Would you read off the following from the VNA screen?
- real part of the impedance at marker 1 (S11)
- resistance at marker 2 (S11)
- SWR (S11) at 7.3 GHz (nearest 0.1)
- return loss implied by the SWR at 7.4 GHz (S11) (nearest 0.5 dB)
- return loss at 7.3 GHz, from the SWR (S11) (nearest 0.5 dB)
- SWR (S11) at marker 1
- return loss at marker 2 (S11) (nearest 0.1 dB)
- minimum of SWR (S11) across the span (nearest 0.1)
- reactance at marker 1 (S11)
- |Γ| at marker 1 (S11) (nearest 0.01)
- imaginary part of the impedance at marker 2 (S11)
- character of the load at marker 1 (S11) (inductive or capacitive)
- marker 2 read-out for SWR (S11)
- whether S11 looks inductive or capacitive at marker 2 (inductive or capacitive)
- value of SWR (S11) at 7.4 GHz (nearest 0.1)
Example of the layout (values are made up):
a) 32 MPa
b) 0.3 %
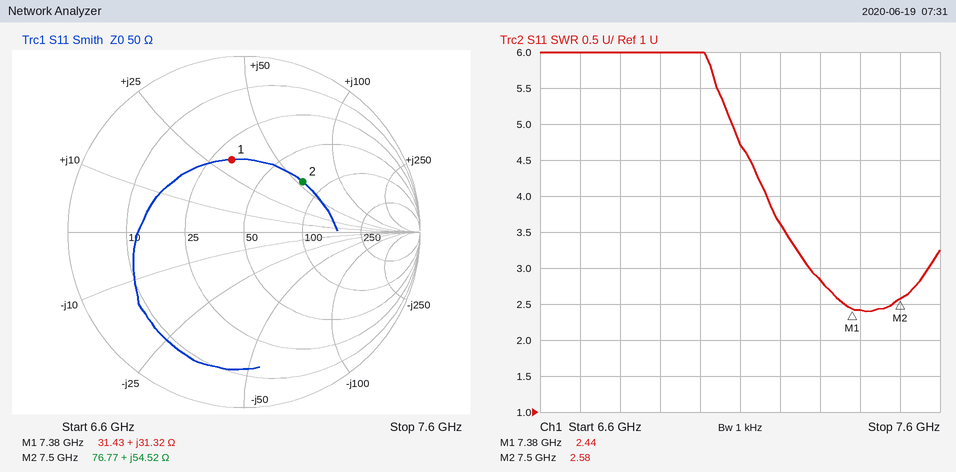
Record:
a) 31.43 Ω
b) 76.77 Ω
c) 2.8
d) 7.5 dB
e) 6.5 dB
f) 2.44
g) 7.1 dB
h) 2.4
i) +31.32 Ω
j) 0.42
k) +54.52 Ω
l) inductive
m) 2.58
n) inductive
o) 2.4
